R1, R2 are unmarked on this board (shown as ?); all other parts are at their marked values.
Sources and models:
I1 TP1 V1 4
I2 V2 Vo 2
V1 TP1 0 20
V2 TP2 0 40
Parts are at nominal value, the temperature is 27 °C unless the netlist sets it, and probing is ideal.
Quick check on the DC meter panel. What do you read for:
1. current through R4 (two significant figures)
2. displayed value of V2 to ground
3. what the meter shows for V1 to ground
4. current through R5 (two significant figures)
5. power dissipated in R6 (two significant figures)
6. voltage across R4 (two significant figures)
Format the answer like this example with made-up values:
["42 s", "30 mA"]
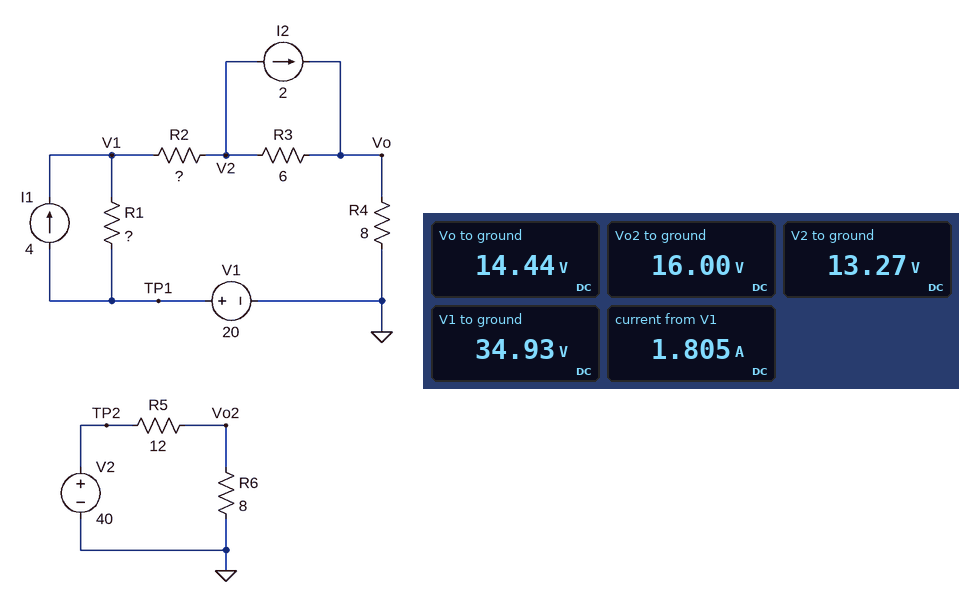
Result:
["1.8 A", "13.27 V", "34.93 V", "2.0 A", "32 W", "14 V"]
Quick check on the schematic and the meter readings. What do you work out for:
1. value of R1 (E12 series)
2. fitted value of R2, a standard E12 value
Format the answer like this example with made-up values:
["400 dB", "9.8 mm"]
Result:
["6.8 Ω", "12 Ω"]
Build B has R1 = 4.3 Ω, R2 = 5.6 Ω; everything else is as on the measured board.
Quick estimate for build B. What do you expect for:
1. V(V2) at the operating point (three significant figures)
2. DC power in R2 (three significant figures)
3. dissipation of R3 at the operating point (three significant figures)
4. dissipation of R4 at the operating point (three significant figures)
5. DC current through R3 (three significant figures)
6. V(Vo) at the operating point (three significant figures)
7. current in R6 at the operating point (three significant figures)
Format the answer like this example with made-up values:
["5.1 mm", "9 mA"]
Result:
["16.8 V", "23.7 W", "20.6 mW", "33.9 W", "58.6 mA", "16.5 V", "2.00 A"]
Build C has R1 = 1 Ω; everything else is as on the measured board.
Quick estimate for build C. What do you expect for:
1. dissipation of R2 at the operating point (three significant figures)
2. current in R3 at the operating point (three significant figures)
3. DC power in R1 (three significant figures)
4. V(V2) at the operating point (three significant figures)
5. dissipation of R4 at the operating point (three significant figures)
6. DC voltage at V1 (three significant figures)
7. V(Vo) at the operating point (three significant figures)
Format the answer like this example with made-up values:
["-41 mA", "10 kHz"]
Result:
["21.3 W", "667 mA", "7.11 W", "6.67 V", "14.2 W", "22.7 V", "10.7 V"]
